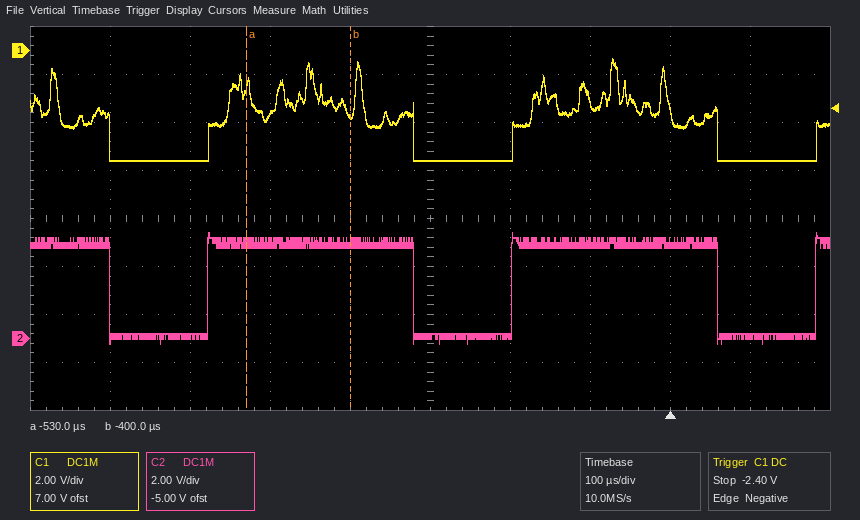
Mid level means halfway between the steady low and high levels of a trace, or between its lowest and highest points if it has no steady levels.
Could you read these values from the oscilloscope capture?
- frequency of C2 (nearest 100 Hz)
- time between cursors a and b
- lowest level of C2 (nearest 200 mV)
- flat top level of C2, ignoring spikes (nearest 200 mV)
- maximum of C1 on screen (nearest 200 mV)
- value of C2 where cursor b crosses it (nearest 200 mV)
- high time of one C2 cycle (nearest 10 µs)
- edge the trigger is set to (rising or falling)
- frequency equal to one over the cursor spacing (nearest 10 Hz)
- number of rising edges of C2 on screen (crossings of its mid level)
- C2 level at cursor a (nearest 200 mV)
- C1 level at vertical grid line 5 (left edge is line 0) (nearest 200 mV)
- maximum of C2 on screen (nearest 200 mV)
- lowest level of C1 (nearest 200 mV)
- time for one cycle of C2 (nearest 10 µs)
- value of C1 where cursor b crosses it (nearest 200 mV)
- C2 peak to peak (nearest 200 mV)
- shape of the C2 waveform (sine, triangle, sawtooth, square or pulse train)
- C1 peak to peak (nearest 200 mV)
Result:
2.6 kHz
130 µs
-200 mV
4.0 V
-400 mV
4.0 V
260 µs
falling
7.69 kHz
3
4.0 V
-4.6 V
4.4 V
-4.6 V
380 µs
-2.6 V
4.6 V
pulse train
4.2 V
